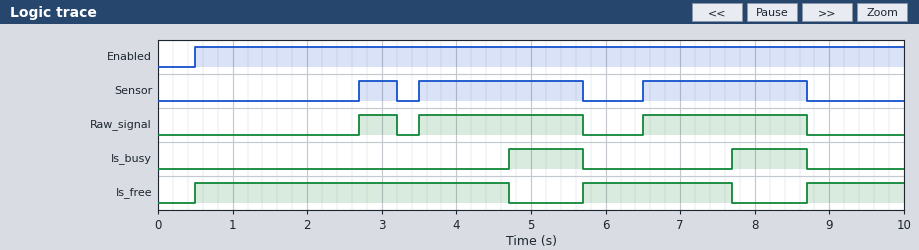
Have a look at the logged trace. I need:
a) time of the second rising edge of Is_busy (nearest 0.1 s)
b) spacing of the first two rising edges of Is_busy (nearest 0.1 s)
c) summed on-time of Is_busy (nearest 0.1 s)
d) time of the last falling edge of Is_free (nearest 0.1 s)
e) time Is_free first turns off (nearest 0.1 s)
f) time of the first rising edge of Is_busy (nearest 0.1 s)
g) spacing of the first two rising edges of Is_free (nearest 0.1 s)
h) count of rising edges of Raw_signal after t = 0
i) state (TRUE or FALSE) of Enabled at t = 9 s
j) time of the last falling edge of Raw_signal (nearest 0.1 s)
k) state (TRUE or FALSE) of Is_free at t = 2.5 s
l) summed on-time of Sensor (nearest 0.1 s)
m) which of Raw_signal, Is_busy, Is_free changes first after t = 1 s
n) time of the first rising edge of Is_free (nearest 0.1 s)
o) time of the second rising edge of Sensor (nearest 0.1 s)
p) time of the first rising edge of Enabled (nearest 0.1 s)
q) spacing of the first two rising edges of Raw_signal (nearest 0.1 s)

7.7 s
3.0 s
2.0 s
7.7 s
4.7 s
4.7 s
5.2 s
3
TRUE
8.7 s
TRUE
4.9 s
Raw_signal
0.5 s
3.5 s
0.5 s
0.8 s
